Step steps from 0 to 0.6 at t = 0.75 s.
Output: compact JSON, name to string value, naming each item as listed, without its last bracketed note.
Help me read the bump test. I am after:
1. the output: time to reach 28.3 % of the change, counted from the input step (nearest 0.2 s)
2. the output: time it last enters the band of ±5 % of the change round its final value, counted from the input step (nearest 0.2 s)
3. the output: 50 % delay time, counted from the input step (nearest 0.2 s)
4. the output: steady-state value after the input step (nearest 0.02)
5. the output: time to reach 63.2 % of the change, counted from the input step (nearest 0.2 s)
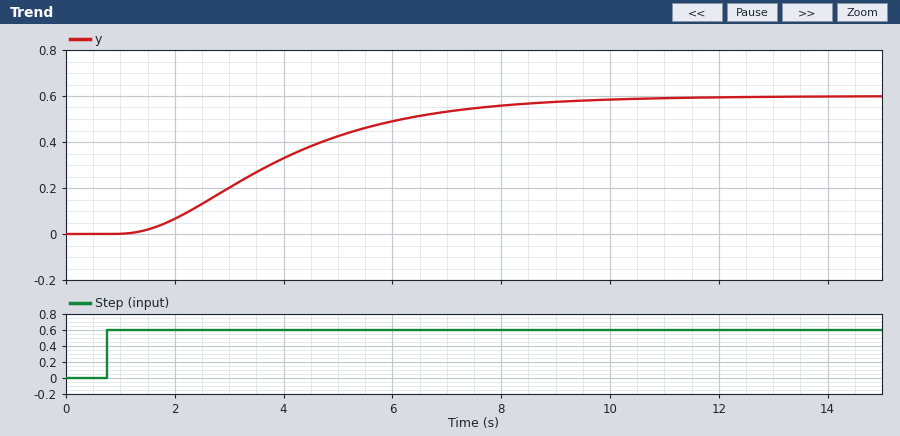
{"the output: time to reach 28.3 % of the change, counted from the input step": "2.0 s", "the output: time it last enters the band of ±5 % of the change round its final value, counted from the input step": "8.0 s", "the output: 50 % delay time, counted from the input step": "3.0 s", "the output: steady-state value after the input step": "0.60", "the output: time to reach 63.2 % of the change, counted from the input step": "3.8 s"}
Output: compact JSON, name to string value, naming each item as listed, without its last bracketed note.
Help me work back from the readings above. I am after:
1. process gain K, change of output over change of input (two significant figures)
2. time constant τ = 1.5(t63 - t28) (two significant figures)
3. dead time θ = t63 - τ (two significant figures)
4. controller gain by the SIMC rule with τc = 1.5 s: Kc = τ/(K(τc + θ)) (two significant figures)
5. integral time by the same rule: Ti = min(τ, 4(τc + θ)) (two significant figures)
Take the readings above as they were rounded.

{"process gain K, change of output over change of input": "1.0", "time constant τ = 1.5(t63 - t28)": "2.7 s", "dead time θ = t63 - τ": "1.1 s", "controller gain by the SIMC rule with τc = 1.5 s: Kc = τ/(K(τc + θ))": "1.0", "integral time by the same rule: Ti = min(τ, 4(τc + θ))": "2.7 s"}
